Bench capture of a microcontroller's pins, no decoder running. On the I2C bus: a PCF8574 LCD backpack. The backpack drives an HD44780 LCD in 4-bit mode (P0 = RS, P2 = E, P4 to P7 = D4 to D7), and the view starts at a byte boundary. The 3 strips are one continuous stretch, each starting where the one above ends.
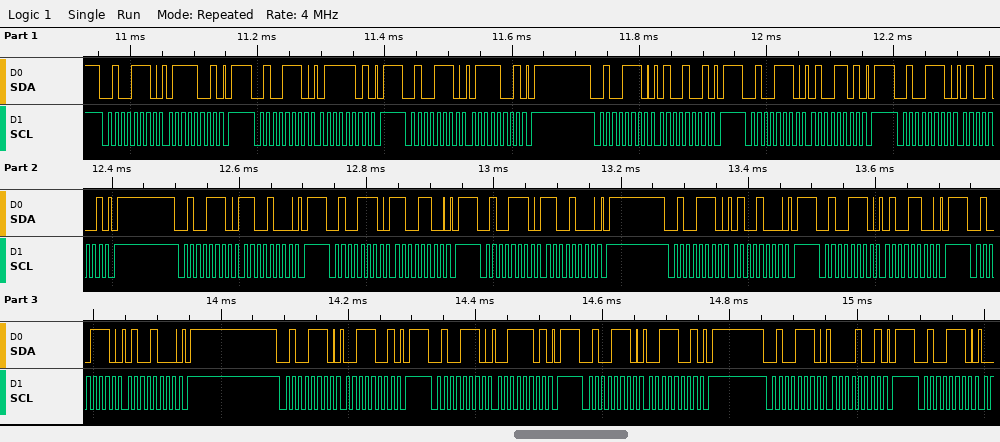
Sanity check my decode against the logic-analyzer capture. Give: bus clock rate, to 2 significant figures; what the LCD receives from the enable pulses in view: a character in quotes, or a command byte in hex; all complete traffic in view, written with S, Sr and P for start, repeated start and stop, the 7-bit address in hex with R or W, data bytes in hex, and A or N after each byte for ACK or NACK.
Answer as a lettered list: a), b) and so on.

a) 100 kHz
b) 't' 0xC4
c) S 27W A 79 A P S 27W A 7D A P S 27W A 79 A P S 27W A 49 A P S 27W A 4D A P S 27W A 49 A P S 27W A C8 A P S 27W A CC A P S 27W A C8 A P S 27W A 48 A P S 27W A 4C A P S 27W A 48 A P S 27W A 39 A P S 27W A 3D A P S 27W A 39 A P S 27W A 09 A P S 27W A
